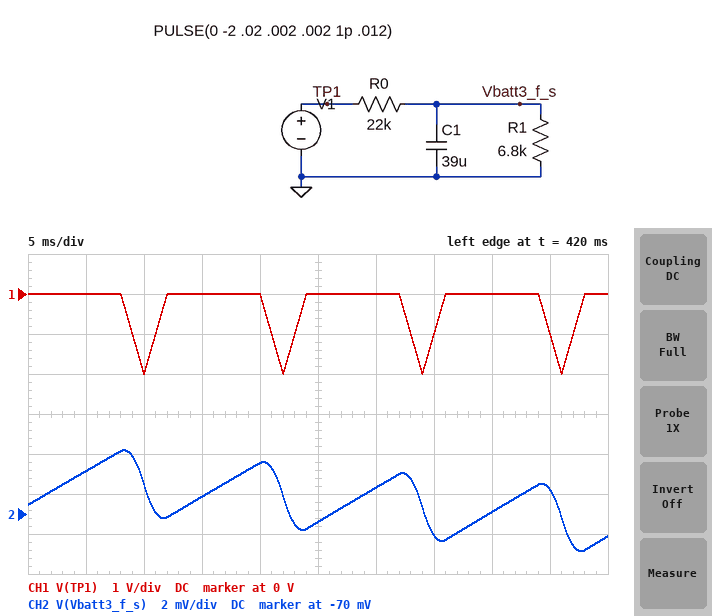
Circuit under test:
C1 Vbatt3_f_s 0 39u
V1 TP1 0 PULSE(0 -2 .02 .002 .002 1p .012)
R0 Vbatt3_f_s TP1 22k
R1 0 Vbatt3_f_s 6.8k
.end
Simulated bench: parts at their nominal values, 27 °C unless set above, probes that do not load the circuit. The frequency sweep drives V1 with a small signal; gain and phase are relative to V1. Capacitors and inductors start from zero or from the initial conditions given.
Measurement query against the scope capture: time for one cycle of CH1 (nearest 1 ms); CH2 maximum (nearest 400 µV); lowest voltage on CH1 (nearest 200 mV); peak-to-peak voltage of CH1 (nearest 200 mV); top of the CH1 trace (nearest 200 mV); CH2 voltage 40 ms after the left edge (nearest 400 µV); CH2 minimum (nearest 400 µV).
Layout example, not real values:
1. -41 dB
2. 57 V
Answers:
1. 12 ms
2. -66.8 mV
3. -2.0 V
4. 2.0 V
5. 0 V
6. -70.0 mV
7. -72.0 mV
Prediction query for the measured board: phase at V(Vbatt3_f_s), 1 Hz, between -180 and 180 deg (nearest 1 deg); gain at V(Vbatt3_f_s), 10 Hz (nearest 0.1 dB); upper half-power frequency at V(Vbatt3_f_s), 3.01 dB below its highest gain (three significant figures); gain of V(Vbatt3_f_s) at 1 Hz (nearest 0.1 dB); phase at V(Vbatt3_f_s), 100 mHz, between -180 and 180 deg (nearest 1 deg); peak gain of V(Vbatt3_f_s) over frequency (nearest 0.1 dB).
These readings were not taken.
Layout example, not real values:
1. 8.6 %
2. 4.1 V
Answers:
1. -52 deg
2. -34.7 dB
3. 786 mHz
4. -16.7 dB
5. -7 deg
6. -12.5 dB
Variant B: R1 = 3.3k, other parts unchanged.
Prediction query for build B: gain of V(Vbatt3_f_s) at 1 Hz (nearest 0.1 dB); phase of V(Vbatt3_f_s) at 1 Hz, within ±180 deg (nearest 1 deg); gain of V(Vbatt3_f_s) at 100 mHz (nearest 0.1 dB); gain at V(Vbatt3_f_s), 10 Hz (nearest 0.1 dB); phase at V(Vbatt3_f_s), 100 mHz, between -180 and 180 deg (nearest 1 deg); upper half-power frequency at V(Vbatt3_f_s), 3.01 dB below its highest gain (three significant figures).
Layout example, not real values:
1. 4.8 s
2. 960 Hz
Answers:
1. -19.4 dB
2. -35 deg
3. -17.7 dB
4. -34.7 dB
5. -4 deg
6. 1.42 Hz
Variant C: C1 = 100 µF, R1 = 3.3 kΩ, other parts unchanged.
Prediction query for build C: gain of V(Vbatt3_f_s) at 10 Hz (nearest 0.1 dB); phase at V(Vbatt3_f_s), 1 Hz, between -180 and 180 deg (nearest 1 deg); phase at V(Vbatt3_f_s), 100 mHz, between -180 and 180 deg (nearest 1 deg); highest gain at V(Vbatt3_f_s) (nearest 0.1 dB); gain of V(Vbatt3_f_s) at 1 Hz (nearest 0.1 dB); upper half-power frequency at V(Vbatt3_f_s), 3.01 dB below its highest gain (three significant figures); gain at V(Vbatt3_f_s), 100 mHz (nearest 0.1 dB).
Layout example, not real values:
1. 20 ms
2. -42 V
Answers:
1. -42.8 dB
2. -61 deg
3. -10 deg
4. -17.7 dB
5. -24.0 dB
6. 555 mHz
7. -17.8 dB
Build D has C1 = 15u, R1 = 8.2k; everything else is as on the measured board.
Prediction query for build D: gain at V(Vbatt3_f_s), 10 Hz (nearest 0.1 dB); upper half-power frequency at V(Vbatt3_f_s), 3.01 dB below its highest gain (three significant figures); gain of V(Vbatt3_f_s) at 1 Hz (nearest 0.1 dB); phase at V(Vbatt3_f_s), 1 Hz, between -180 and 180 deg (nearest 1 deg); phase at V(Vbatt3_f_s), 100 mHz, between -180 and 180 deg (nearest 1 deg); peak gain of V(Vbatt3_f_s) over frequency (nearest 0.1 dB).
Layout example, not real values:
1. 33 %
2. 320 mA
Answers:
1. -26.5 dB
2. 1.78 Hz
3. -12.5 dB
4. -29 deg
5. -3 deg
6. -11.3 dB
